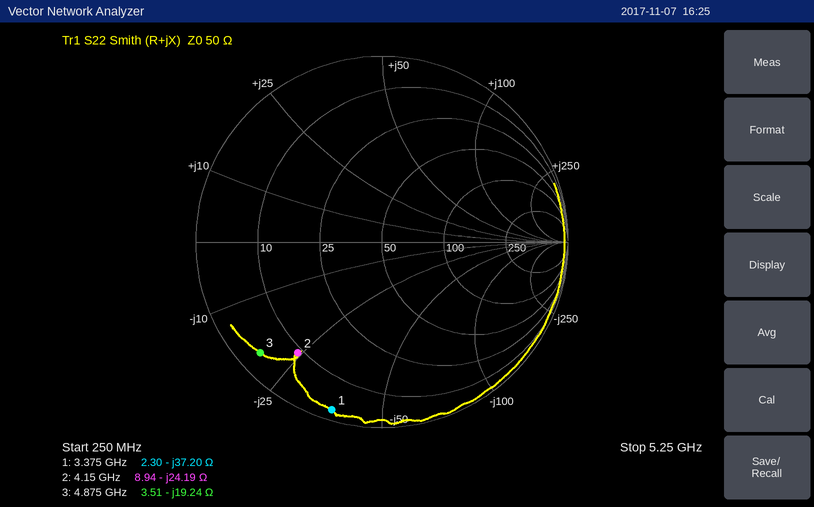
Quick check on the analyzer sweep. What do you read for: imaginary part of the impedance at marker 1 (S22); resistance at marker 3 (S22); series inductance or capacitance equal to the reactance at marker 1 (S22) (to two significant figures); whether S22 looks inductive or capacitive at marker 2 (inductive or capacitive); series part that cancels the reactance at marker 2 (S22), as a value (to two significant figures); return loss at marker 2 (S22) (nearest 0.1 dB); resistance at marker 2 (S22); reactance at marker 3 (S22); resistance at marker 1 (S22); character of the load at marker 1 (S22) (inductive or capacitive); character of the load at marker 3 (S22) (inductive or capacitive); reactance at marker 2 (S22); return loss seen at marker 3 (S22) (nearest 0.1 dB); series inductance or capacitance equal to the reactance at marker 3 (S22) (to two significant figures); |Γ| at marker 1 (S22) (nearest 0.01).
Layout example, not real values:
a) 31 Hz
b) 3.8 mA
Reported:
a) -37.20 Ω
b) 3.51 Ω
c) 1.3 pF
d) capacitive
e) 930 pH
f) 2.5 dB
g) 8.94 Ω
h) -19.24 Ω
i) 2.30 Ω
j) capacitive
k) capacitive
l) -24.19 Ω
m) 1.1 dB
n) 1.7 pF
o) 0.94
